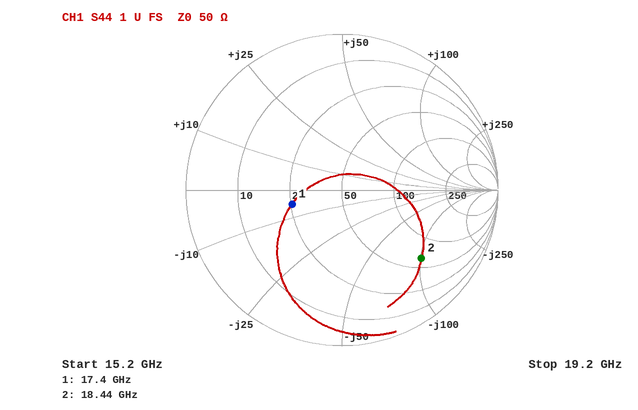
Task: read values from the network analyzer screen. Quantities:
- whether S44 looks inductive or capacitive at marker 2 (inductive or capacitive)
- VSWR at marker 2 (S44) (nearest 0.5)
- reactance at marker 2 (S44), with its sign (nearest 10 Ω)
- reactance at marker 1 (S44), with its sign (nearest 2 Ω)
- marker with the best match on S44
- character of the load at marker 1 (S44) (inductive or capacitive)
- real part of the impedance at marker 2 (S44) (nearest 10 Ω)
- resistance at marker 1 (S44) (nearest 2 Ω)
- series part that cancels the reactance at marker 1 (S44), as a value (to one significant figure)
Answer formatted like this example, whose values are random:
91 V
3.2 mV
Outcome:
capacitive
5.0
-100 Ω
-6 Ω
marker 1
capacitive
60 Ω
26 Ω
50 pH
